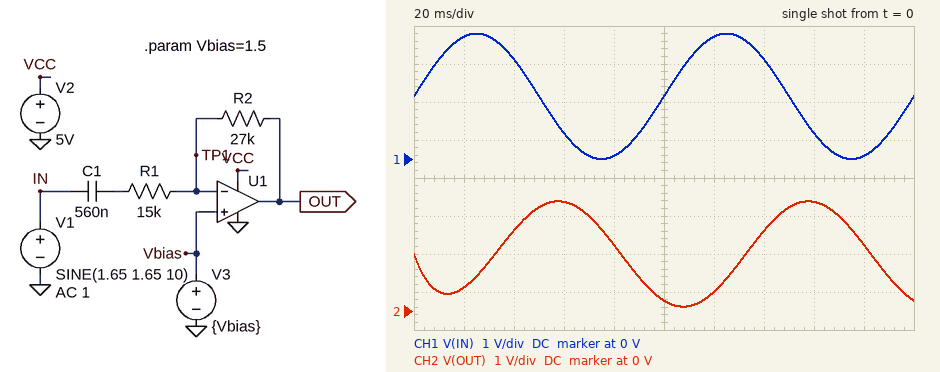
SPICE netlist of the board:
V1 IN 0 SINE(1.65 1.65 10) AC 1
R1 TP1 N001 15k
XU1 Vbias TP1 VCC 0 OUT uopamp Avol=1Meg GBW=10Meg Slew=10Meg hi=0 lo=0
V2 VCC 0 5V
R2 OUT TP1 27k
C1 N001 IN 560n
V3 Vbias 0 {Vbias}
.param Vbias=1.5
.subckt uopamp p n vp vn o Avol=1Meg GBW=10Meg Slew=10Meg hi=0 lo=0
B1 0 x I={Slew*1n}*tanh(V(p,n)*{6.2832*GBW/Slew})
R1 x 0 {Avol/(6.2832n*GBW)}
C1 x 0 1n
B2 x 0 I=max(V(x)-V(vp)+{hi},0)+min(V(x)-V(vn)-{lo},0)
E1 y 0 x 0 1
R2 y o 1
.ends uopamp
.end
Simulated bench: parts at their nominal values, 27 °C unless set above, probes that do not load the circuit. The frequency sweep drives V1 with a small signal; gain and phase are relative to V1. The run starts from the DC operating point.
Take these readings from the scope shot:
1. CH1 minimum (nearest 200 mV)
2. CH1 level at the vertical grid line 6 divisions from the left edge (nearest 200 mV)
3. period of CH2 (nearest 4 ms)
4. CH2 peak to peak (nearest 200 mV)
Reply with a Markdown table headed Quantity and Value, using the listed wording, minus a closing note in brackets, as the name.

| Quantity | Value |
|---|---|
| CH1 minimum | 0 V |
| CH1 level at the vertical grid line 6 divisions from the left edge | 3.2 V |
| period of CH2 | 100 ms |
| CH2 peak to peak | 2.8 V |
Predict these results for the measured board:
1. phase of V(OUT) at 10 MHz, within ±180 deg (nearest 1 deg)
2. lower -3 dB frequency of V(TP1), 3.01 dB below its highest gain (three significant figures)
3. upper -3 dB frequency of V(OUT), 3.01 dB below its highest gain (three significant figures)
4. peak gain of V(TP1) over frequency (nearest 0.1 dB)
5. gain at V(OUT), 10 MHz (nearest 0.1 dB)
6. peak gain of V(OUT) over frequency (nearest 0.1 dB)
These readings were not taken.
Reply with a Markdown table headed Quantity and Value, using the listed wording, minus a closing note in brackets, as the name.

| Quantity | Value |
|---|---|
| phase of V(OUT) at 10 MHz, within ±180 deg | 110 deg |
| lower -3 dB frequency of V(TP1), 3.01 dB below its highest gain | 3.57 MHz |
| upper -3 dB frequency of V(OUT), 3.01 dB below its highest gain | 3.57 MHz |
| peak gain of V(TP1) over frequency | -3.8 dB |
| gain at V(OUT), 10 MHz | -4.4 dB |
| peak gain of V(OUT) over frequency | 5.1 dB |
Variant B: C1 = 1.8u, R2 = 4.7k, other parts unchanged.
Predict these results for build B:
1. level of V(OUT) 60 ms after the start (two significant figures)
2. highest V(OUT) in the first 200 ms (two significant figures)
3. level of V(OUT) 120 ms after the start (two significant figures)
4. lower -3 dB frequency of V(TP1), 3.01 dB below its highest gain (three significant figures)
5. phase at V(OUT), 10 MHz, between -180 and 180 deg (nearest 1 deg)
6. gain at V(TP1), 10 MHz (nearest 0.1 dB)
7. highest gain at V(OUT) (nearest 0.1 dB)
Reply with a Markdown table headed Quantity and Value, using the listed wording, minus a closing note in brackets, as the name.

| Quantity | Value |
|---|---|
| level of V(OUT) 60 ms after the start | 1.9 V |
| highest V(OUT) in the first 200 ms | 2.0 V |
| level of V(OUT) 120 ms after the start | 1.1 V |
| lower -3 dB frequency of V(TP1), 3.01 dB below its highest gain | 7.61 MHz |
| phase at V(OUT), 10 MHz, between -180 and 180 deg | 127 deg |
| gain at V(TP1), 10 MHz | -14.4 dB |
| highest gain at V(OUT) | -10.1 dB |
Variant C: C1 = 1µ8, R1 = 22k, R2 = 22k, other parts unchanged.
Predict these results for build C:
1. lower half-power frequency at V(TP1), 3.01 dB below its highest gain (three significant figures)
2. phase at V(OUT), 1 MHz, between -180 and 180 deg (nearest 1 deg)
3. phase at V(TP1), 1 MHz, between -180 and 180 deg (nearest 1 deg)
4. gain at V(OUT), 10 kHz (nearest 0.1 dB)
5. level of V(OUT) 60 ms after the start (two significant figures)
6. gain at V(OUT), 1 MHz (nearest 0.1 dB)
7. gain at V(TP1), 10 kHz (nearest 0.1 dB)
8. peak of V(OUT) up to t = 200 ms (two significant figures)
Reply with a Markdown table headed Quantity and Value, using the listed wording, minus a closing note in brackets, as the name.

| Quantity | Value |
|---|---|
| lower half-power frequency at V(TP1), 3.01 dB below its highest gain | 5.00 MHz |
| phase at V(OUT), 1 MHz, between -180 and 180 deg | 169 deg |
| phase at V(TP1), 1 MHz, between -180 and 180 deg | 79 deg |
| gain at V(OUT), 10 kHz | 0 dB |
| level of V(OUT) 60 ms after the start | 2.9 V |
| gain at V(OUT), 1 MHz | -0.2 dB |
| gain at V(TP1), 10 kHz | -60.0 dB |
| peak of V(OUT) up to t = 200 ms | 3.1 V |
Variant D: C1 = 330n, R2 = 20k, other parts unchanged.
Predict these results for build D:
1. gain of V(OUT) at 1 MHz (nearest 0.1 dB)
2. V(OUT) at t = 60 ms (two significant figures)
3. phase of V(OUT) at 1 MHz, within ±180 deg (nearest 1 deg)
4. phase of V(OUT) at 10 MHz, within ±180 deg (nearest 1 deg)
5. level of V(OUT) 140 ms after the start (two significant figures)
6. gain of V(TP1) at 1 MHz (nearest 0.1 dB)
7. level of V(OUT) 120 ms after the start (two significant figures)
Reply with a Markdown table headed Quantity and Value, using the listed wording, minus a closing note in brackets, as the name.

| Quantity | Value |
|---|---|
| gain of V(OUT) at 1 MHz | 2.3 dB |
| V(OUT) at t = 60 ms | 2.1 V |
| phase of V(OUT) at 1 MHz, within ±180 deg | 167 deg |
| phase of V(OUT) at 10 MHz, within ±180 deg | 113 deg |
| level of V(OUT) 140 ms after the start | 1.9 V |
| gain of V(TP1) at 1 MHz | -17.7 dB |
| level of V(OUT) 120 ms after the start | 1.1 V |
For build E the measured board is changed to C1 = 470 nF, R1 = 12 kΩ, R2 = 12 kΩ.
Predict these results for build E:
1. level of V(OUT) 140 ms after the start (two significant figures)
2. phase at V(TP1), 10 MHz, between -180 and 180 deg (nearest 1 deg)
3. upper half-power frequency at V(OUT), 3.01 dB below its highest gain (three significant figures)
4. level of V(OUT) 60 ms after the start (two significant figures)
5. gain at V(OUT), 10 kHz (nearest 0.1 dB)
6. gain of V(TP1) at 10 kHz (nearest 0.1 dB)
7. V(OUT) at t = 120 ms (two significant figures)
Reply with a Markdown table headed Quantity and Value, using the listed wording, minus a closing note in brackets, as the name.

| Quantity | Value |
|---|---|
| level of V(OUT) 140 ms after the start | 1.8 V |
| phase at V(TP1), 10 MHz, between -180 and 180 deg | 27 deg |
| upper half-power frequency at V(OUT), 3.01 dB below its highest gain | 5.00 MHz |
| level of V(OUT) 60 ms after the start | 2.0 V |
| gain at V(OUT), 10 kHz | 0 dB |
| gain of V(TP1) at 10 kHz | -60.0 dB |
| V(OUT) at t = 120 ms | 1.2 V |
